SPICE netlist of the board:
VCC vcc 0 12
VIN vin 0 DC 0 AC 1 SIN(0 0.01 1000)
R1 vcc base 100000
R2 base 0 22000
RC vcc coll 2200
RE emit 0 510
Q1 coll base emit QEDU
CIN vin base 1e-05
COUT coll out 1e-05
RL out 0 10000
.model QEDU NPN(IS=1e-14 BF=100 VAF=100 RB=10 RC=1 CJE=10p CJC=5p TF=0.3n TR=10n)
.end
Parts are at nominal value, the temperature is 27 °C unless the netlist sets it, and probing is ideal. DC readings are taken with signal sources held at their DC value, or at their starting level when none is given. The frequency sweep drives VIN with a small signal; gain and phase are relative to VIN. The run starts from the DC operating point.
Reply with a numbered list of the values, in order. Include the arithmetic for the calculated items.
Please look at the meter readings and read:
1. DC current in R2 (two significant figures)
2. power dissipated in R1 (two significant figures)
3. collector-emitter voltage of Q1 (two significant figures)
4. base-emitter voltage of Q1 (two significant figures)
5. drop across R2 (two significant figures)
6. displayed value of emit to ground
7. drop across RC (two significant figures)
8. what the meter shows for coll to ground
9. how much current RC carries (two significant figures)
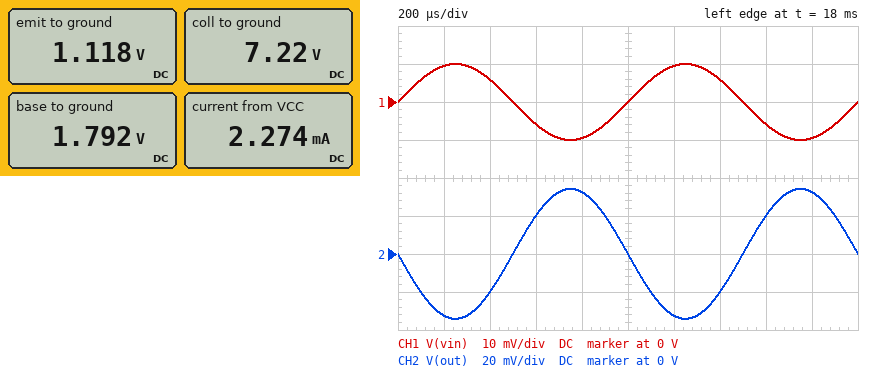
1. (1.792 V) / 22 kΩ = 81 µA
2. (12 V - 1.792 V)^2 / 100 kΩ = 1.0 mW
3. 7.22 V - 1.118 V = 6.1 V
4. 1.792 V - 1.118 V = 670 mV
5. 1.792 V = 1.8 V
6. 1.118 V
7. 12 V - 7.22 V = 4.8 V
8. 7.22 V
9. (12 V - 7.22 V) / 2.2 kΩ = 2.2 mA
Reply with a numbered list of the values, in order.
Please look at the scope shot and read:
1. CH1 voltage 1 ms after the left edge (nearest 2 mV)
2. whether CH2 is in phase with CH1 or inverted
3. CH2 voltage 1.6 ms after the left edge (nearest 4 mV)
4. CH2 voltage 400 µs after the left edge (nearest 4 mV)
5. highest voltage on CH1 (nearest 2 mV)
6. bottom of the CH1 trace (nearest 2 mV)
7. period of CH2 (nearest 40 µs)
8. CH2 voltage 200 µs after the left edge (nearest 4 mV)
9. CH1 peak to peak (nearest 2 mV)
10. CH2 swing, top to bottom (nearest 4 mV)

1. 0 V
2. inverted
3. 20 mV
4. -20 mV
5. 10 mV
6. -10 mV
7. 1.00 ms
8. -32 mV
9. 20 mV
10. 68 mV
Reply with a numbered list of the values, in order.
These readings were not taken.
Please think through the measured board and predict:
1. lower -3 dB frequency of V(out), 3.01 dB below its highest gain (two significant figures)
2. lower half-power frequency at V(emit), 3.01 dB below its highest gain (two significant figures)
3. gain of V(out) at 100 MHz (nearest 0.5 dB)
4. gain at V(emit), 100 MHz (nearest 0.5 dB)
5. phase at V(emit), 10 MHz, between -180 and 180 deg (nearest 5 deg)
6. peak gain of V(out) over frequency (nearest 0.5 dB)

1. 1.9 Hz
2. 1.2 Hz
3. 4.0 dB
4. -0.5 dB
5. 0 deg
6. 10.5 dB
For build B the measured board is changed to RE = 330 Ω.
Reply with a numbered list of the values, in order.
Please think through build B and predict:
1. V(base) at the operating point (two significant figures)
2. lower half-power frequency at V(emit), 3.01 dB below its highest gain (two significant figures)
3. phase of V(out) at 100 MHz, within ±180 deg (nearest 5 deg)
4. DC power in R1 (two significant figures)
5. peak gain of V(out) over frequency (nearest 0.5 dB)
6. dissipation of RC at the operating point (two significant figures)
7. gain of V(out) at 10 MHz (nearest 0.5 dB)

1. 1.7 V
2. 1.4 Hz
3. 65 deg
4. 1.1 mW
5. 14.5 dB
6. 19 mW
7. 14.0 dB
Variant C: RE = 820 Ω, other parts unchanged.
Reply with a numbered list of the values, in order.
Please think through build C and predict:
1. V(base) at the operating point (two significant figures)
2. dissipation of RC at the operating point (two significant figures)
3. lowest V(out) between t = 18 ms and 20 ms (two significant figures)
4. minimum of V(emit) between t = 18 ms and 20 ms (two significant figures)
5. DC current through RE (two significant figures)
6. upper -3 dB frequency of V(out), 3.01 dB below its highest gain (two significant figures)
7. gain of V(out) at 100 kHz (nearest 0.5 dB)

1. 1.9 V
2. 5.0 mW
3. -21 mV
4. 1.2 V
5. 1.5 mA
6. 60 MHz
7. 6.5 dB
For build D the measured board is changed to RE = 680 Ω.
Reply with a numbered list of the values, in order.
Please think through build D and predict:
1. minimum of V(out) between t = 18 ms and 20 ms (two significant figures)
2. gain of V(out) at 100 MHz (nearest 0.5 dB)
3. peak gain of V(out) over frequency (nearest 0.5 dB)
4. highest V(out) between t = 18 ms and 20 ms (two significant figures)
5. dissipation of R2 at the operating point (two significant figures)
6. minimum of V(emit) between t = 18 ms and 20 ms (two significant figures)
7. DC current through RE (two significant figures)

1. -26 mV
2. 3.0 dB
3. 8.0 dB
4. 26 mV
5. 160 µW
6. 1.2 V
7. 1.8 mA
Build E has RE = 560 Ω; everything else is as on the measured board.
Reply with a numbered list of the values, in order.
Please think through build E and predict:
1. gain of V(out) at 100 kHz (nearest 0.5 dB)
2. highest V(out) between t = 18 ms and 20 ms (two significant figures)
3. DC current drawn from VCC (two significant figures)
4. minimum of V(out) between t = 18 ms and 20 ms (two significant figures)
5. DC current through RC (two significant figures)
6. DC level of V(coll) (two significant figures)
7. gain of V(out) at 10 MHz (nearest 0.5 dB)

1. 10.0 dB
2. 31 mV
3. 2.1 mA
4. -31 mV
5. 2.0 mA
6. 7.5 V
7. 9.5 dB
